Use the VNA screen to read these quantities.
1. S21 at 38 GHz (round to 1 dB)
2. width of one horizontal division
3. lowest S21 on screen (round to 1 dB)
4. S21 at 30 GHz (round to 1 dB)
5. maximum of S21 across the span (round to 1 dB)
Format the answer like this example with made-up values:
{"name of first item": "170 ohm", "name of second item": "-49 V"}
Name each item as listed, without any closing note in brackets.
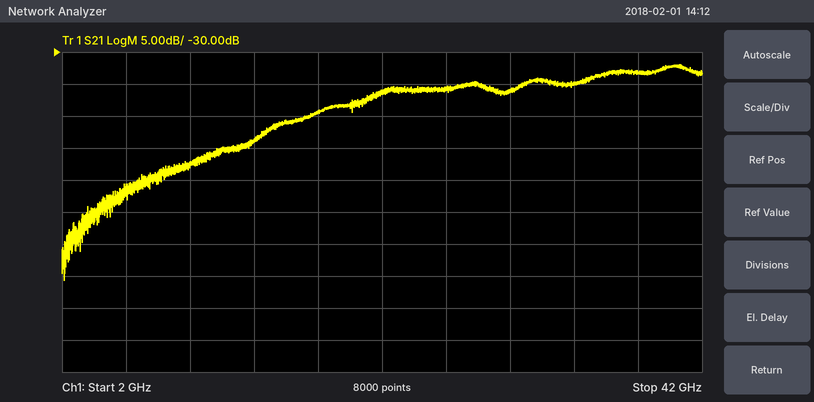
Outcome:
{"S21 at 38 GHz": "-33 dB", "width of one horizontal division": "4 GHz", "lowest S21 on screen": "-66 dB", "S21 at 30 GHz": "-36 dB", "maximum of S21 across the span": "-32 dB"}
